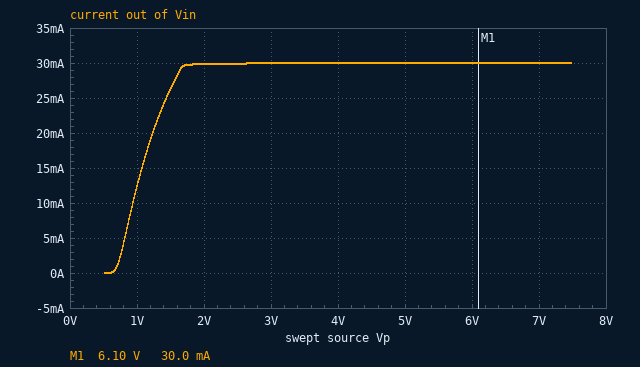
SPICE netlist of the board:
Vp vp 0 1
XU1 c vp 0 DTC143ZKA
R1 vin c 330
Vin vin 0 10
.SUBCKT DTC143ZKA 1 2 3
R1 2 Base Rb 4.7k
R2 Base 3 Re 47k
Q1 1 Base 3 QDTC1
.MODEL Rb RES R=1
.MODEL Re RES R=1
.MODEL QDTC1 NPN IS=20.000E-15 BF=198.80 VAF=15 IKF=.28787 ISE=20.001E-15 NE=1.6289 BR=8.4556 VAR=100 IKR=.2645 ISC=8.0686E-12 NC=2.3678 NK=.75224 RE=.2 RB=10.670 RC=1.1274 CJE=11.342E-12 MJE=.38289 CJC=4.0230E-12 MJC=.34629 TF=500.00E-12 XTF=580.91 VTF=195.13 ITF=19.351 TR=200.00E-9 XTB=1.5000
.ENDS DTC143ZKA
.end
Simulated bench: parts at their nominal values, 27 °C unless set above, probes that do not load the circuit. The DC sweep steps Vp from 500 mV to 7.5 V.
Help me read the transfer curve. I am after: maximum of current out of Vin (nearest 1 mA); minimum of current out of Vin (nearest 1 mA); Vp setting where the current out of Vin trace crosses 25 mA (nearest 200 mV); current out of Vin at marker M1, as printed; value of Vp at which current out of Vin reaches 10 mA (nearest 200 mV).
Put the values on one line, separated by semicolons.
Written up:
30 mA; 0 A; 1.4 V; 30.0 mA; 1.0 V
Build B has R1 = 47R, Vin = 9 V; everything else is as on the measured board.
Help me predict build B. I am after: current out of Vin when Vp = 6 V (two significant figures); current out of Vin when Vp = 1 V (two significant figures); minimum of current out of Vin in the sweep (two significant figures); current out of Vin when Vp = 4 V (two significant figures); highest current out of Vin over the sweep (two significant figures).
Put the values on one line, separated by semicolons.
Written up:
130 mA; 14 mA; 1.3 µA; 100 mA; 140 mA
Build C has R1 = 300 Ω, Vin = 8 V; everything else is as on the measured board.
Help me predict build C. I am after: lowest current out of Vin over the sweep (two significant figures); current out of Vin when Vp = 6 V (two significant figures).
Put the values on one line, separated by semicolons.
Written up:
1.3 µA; 26 mA
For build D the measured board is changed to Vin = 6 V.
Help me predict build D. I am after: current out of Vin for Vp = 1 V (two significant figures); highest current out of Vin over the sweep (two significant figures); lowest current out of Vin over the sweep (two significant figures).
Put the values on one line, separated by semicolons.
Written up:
10 mA; 18 mA; 1.2 µA
